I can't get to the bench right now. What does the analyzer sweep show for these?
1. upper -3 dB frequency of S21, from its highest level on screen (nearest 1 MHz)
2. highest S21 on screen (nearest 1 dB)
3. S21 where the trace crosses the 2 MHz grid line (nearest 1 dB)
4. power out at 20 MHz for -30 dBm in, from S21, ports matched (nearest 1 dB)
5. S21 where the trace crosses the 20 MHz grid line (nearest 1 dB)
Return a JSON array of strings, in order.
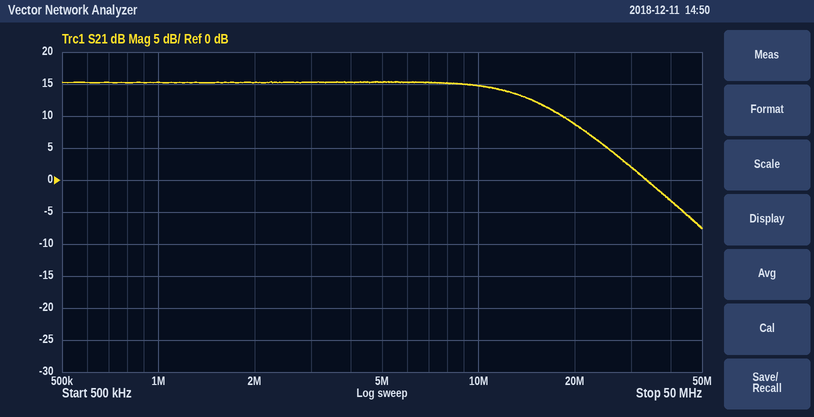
["15 MHz", "15 dB", "15 dB", "-21 dBm", "9 dB"]
